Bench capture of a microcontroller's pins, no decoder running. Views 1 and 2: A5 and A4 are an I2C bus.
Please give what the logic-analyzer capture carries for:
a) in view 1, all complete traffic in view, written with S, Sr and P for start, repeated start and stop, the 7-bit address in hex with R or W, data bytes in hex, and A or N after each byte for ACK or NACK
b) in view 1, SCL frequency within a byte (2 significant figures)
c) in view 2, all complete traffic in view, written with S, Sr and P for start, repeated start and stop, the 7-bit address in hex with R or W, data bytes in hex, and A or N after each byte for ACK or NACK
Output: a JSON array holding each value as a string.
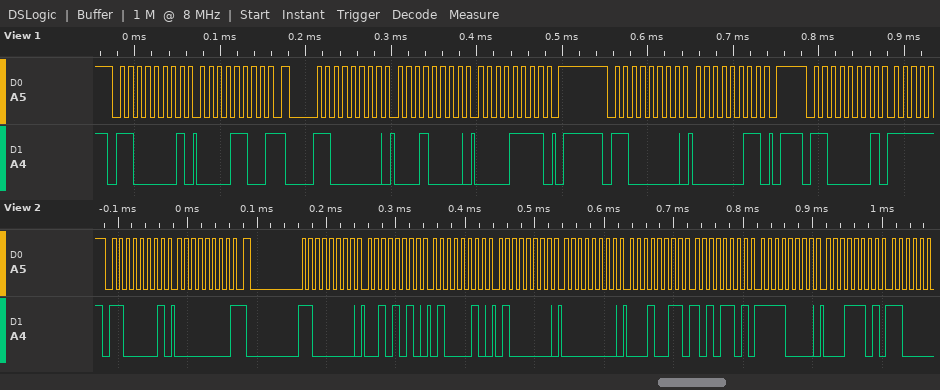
["S 60R A 0C N Sr 60W A 10 A 0F A P S 60W A 03 A P S 60R A", "100 kHz", "S 60R A 00 N Sr 60W A 2A A 42 A 40 A 00 A 13 A AD A F0 A 1D A"]
